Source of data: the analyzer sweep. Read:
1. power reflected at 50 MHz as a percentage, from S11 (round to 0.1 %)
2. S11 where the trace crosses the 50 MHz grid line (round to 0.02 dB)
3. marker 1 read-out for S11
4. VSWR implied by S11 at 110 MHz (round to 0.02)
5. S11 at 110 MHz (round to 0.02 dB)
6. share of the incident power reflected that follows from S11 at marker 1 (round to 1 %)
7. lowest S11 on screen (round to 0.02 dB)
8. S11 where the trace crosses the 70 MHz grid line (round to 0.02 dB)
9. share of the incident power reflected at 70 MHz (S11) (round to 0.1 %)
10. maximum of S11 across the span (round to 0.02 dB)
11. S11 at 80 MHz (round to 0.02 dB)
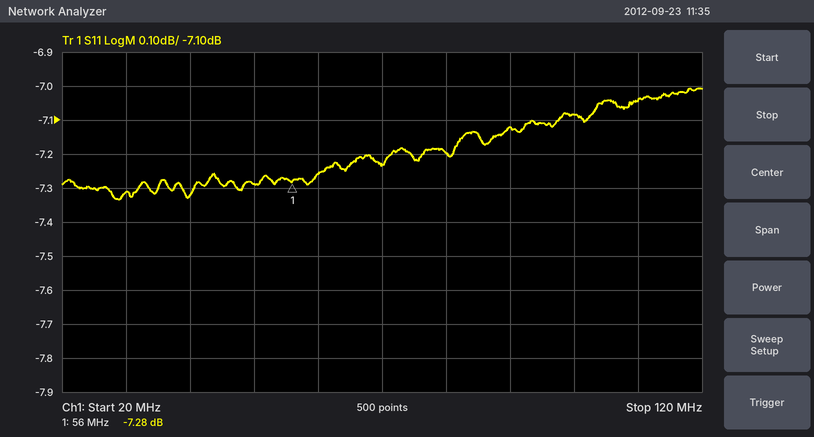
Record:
18.7 %
-7.28 dB
-7.28 dB
2.60
-7.04 dB
19 %
-7.34 dB
-7.24 dB
18.9 %
-7.00 dB
-7.20 dB
